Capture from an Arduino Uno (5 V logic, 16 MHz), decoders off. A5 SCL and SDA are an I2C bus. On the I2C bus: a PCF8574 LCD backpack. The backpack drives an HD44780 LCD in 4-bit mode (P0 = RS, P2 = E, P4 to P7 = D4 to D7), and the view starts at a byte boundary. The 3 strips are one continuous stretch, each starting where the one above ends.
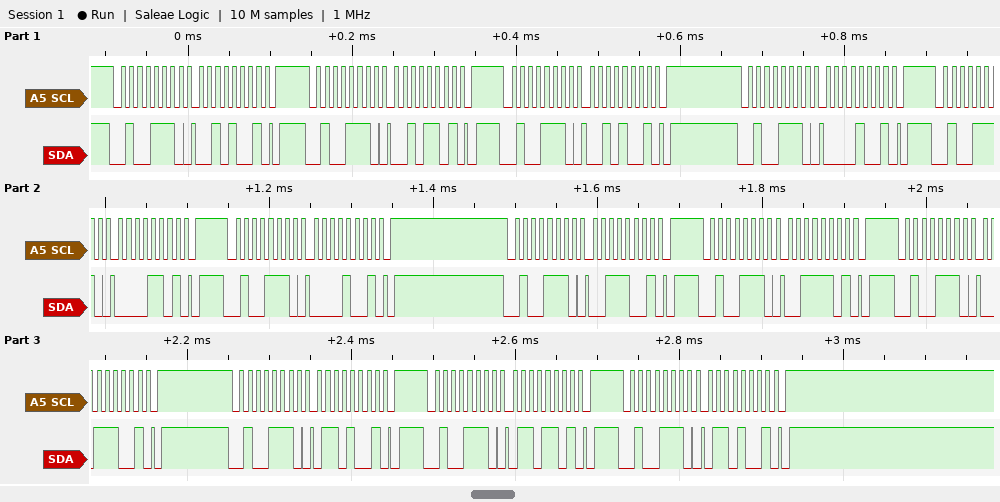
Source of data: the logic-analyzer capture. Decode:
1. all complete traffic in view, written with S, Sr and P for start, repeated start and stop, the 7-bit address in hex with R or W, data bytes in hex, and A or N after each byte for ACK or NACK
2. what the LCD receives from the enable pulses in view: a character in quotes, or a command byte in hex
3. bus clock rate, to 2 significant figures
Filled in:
S 27W A 29 A P S 27W A 2D A P S 27W A 29 A P S 27W A 09 A P S 27W A 0D A P S 27W A 09 A P S 27W A 39 A P S 27W A 3D A P S 27W A 39 A P S 27W A 69 A P S 27W A 6D A P S 27W A 69 A P
' ' '6'
100 kHz
